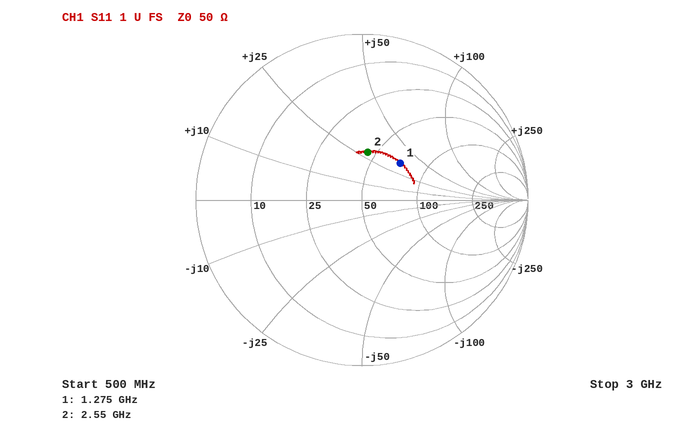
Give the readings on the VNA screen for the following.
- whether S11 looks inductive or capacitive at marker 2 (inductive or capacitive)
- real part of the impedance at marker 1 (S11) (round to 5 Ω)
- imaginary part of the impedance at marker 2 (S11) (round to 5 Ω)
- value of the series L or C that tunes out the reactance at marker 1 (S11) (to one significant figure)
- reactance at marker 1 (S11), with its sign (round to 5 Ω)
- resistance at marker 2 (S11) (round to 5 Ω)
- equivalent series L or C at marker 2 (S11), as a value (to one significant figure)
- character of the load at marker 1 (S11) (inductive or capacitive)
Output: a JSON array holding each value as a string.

["inductive", "70 Ω", "+30 Ω", "4 pF", "+35 Ω", "45 Ω", "2 nH", "inductive"]
